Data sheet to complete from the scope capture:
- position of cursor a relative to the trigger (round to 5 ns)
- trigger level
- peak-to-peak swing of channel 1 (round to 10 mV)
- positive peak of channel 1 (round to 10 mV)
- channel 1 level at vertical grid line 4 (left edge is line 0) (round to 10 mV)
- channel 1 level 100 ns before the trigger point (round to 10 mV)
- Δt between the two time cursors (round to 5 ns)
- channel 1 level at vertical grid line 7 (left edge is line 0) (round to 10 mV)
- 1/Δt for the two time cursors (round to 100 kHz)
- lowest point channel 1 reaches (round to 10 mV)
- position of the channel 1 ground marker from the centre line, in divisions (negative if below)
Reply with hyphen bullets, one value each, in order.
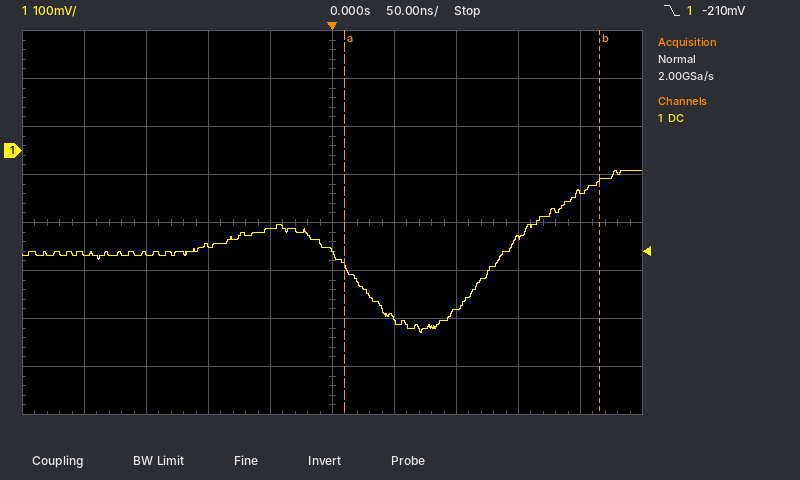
- +10 ns
- -210 mV
- 340 mV
- -40 mV
- -160 mV
- -200 mV
- 205 ns
- -330 mV
- 4.9 MHz
- -380 mV
- +1.5 div
